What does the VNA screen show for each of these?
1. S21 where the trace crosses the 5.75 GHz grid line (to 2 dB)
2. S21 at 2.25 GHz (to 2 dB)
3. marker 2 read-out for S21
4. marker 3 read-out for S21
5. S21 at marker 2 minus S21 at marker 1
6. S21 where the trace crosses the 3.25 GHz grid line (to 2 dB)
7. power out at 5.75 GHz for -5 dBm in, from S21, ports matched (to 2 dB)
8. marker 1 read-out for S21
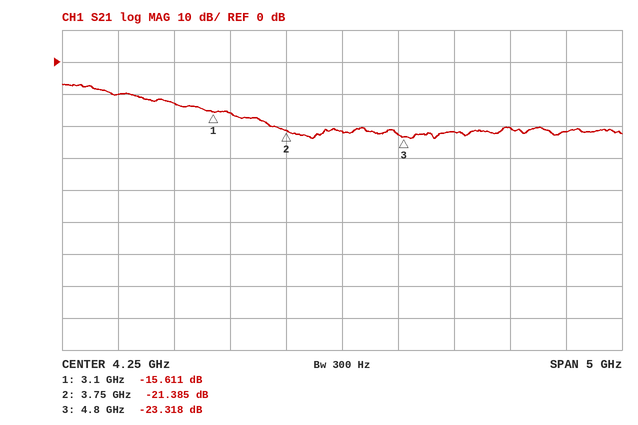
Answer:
-20 dB
-10 dB
-21.385 dB
-23.318 dB
-5.774 dB
-16 dB
-26 dBm
-15.611 dB
